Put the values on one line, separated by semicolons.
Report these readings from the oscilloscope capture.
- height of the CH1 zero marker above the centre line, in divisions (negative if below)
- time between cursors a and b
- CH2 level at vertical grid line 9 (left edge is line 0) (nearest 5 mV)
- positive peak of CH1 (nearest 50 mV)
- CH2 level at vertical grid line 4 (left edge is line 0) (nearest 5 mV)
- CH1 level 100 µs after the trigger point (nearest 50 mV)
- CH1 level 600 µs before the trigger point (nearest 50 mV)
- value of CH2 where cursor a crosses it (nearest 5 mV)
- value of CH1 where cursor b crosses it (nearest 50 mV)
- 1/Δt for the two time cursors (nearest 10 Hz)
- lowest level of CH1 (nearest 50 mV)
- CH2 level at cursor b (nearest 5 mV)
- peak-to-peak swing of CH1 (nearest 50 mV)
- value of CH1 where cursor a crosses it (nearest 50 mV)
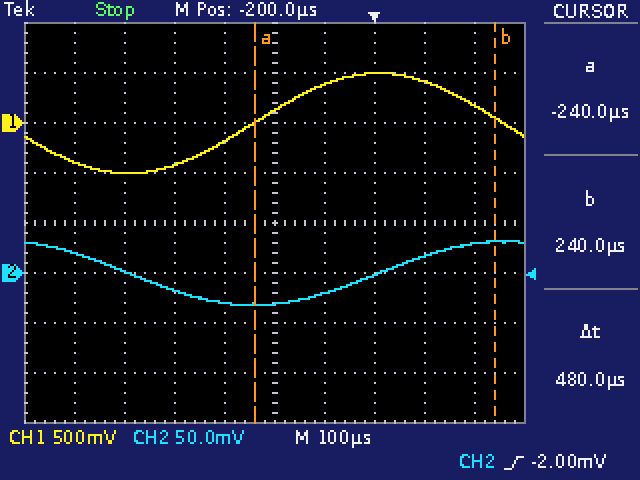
+2.0 div; 480 µs; 30 mV; 500 mV; -30 mV; 400 mV; -400 mV; -30 mV; 50 mV; 2.08 kHz; -500 mV; 30 mV; 1.00 V; 0 mV
